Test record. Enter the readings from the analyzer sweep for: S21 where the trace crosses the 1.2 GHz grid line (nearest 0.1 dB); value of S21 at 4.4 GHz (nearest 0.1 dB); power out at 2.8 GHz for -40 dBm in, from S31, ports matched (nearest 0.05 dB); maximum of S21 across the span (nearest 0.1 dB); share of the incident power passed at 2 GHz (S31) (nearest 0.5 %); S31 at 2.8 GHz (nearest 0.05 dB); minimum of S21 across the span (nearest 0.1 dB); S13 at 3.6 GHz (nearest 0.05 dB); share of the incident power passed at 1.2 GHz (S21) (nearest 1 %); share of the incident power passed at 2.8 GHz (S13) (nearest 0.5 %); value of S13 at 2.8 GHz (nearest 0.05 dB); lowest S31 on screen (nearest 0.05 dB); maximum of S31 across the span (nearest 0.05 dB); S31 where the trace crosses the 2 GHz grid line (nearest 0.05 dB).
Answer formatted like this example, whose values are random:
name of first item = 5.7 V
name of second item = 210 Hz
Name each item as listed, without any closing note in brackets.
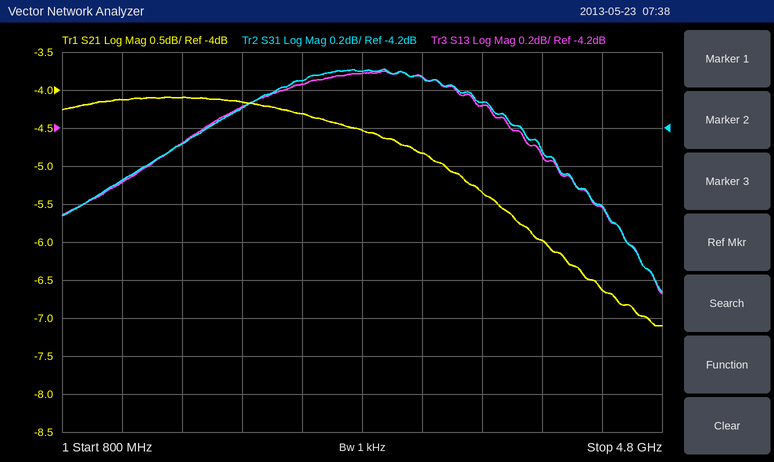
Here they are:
S21 where the trace crosses the 1.2 GHz grid line = -4.1 dB
value of S21 at 4.4 GHz = -6.6 dB
power out at 2.8 GHz for -40 dBm in, from S31, ports matched = -43.90 dBm
maximum of S21 across the span = -4.1 dB
share of the incident power passed at 2 GHz (S31) = 39.0 %
S31 at 2.8 GHz = -3.90 dB
minimum of S21 across the span = -7.1 dB
S13 at 3.6 GHz = -4.10 dB
share of the incident power passed at 1.2 GHz (S21) = 39 %
share of the incident power passed at 2.8 GHz (S13) = 40.5 %
value of S13 at 2.8 GHz = -3.90 dB
lowest S31 on screen = -5.05 dB
maximum of S31 across the span = -3.90 dB
S31 where the trace crosses the 2 GHz grid line = -4.10 dB
